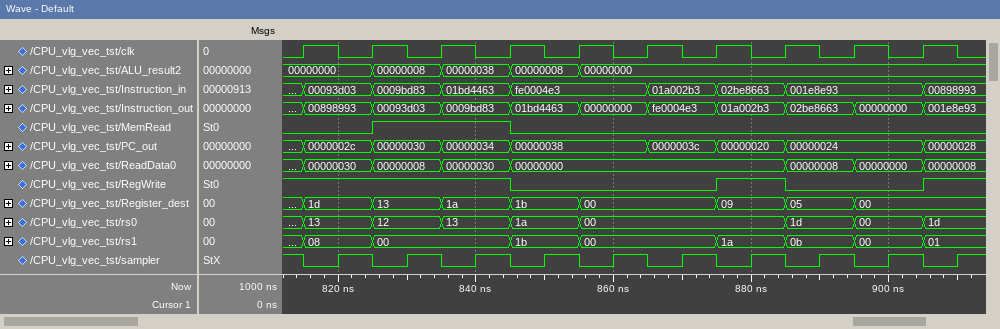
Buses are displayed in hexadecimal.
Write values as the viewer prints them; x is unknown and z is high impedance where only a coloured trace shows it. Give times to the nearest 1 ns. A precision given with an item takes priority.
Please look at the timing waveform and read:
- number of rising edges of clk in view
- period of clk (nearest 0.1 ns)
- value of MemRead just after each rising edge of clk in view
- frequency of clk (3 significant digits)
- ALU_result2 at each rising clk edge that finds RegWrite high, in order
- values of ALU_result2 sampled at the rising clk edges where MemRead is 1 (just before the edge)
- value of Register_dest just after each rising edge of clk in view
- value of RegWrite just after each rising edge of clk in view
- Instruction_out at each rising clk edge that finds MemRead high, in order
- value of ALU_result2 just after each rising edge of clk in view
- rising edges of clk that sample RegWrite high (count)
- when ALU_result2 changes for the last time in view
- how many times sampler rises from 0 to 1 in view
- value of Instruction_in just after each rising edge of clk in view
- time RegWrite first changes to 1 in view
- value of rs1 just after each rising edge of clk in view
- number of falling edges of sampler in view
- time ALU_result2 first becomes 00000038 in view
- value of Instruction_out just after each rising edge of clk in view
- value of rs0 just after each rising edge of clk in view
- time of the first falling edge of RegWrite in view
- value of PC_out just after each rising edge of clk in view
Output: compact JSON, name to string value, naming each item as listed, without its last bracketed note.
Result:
{"number of rising edges of clk in view": "10", "period of clk": "10 ns", "value of MemRead just after each rising edge of clk in view": "0 1 1 0 0 0 0 0 0 0", "frequency of clk": "100 MHz", "ALU_result2 at each rising clk edge that finds RegWrite high, in order": "00000000, 00000000, 00000008, 00000038, 00000000", "values of ALU_result2 sampled at the rising clk edges where MemRead is 1": "00000008, 00000038", "value of Register_dest just after each rising edge of clk in view": "1d, 13, 1a, 1b, 00, 00, 09, 05, 00, 00", "value of RegWrite just after each rising edge of clk in view": "1 1 1 0 0 0 1 0 0 1", "Instruction_out at each rising clk edge that finds MemRead high, in order": "00093d03, 0009bd83", "value of ALU_result2 just after each rising edge of clk in view": "00000000, 00000008, 00000038, 00000008, 00000000, 00000000, 00000000, 00000000, 00000000, 00000000", "rising edges of clk that sample RegWrite high": "5", "when ALU_result2 changes for the last time in view": "855 ns", "how many times sampler rises from 0 to 1 in view": "10", "value of Instruction_in just after each rising edge of clk in view": "00093d03, 0009bd83, 01bd4463, fe0004e3, fe0004e3, 01a002b3, 02be8663, 001e8e93, 001e8e93, 00898993", "time RegWrite first changes to 1 in view": "875 ns", "value of rs1 just after each rising edge of clk in view": "08, 00, 00, 1b, 00, 00, 1a, 0b, 00, 01", "number of falling edges of sampler in view": "10", "time ALU_result2 first becomes 00000038 in view": "835 ns", "value of Instruction_out just after each rising edge of clk in view": "00898993, 00093d03, 0009bd83, 01bd4463, 00000000, fe0004e3, 01a002b3, 02be8663, 00000000, 001e8e93", "value of rs0 just after each rising edge of clk in view": "13, 12, 13, 1a, 00, 00, 00, 1d, 00, 1d", "time of the first falling edge of RegWrite in view": "845 ns", "value of PC_out just after each rising edge of clk in view": "0000002c, 00000030, 00000034, 00000038, 00000038, 0000003c, 00000020, 00000024, 00000024, 00000028"}
